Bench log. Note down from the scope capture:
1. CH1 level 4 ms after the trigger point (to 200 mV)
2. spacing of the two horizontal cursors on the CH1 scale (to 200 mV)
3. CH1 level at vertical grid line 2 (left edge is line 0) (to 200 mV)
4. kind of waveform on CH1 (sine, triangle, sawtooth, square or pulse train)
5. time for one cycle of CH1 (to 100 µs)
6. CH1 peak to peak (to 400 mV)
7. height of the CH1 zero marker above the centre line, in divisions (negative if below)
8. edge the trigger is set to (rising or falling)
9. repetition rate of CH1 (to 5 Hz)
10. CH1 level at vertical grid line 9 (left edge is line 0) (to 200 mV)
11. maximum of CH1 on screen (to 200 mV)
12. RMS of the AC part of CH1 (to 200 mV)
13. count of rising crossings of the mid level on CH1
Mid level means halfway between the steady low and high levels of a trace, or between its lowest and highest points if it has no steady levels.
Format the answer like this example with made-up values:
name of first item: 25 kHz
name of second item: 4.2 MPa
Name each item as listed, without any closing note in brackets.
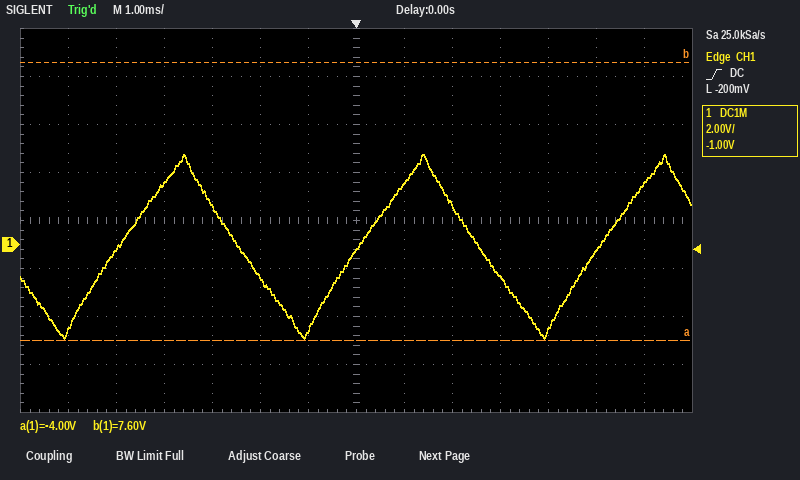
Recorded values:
CH1 level 4 ms after the trigger point: -3.6 V
spacing of the two horizontal cursors on the CH1 scale: 11.6 V
CH1 level at vertical grid line 2 (left edge is line 0): -200 mV
kind of waveform on CH1: triangle
time for one cycle of CH1: 5.0 ms
CH1 peak to peak: 7.6 V
height of the CH1 zero marker above the centre line, in divisions: -0.5 div
edge the trigger is set to: rising
repetition rate of CH1: 200 Hz
CH1 level at vertical grid line 9 (left edge is line 0): 1.6 V
maximum of CH1 on screen: 3.8 V
RMS of the AC part of CH1: 2.2 V
count of rising crossings of the mid level on CH1: 3
